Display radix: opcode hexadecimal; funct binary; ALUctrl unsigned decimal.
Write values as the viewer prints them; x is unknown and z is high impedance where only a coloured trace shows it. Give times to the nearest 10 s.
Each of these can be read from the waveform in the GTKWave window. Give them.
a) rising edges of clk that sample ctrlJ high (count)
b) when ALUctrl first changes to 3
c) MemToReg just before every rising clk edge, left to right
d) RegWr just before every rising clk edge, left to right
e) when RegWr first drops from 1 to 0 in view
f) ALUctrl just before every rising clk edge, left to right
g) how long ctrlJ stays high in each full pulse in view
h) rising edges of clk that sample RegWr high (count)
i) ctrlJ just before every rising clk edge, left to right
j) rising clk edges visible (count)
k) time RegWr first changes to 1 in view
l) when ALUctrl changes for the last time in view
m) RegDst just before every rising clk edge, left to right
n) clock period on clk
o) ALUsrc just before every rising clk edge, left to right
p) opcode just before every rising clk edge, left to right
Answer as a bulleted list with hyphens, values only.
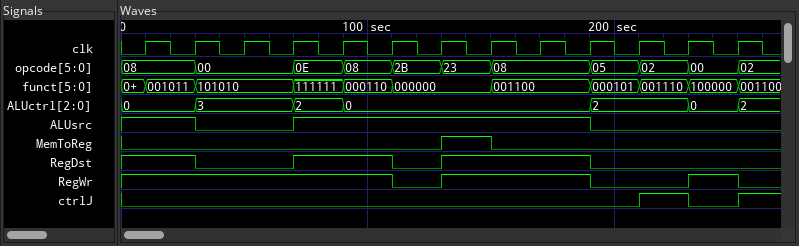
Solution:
- 1
- 30 s
- 0 0 0 0 0 0 0 1 0 0 0 0 0
- 1 1 1 1 1 1 0 1 1 1 0 0 1
- 110 s
- 0, 0, 3, 3, 2, 0, 0, 0, 0, 0, 2, 2, 0
- 20 s
- 10
- 0 0 0 0 0 0 0 0 0 0 0 1 0
- 13
- 130 s
- 250 s
- 1 1 0 0 1 1 0 1 1 1 0 0 0
- 20 s
- 1 1 0 0 1 1 1 1 1 1 0 0 0
- 08, 08, 00, 00, 0E, 08, 2B, 23, 08, 08, 05, 02, 00
